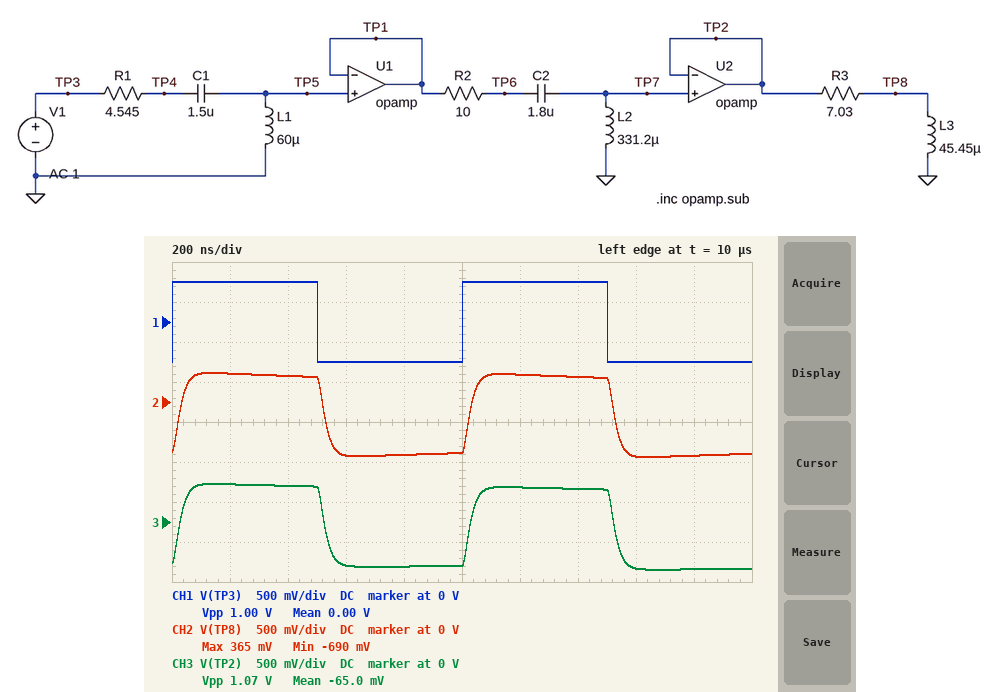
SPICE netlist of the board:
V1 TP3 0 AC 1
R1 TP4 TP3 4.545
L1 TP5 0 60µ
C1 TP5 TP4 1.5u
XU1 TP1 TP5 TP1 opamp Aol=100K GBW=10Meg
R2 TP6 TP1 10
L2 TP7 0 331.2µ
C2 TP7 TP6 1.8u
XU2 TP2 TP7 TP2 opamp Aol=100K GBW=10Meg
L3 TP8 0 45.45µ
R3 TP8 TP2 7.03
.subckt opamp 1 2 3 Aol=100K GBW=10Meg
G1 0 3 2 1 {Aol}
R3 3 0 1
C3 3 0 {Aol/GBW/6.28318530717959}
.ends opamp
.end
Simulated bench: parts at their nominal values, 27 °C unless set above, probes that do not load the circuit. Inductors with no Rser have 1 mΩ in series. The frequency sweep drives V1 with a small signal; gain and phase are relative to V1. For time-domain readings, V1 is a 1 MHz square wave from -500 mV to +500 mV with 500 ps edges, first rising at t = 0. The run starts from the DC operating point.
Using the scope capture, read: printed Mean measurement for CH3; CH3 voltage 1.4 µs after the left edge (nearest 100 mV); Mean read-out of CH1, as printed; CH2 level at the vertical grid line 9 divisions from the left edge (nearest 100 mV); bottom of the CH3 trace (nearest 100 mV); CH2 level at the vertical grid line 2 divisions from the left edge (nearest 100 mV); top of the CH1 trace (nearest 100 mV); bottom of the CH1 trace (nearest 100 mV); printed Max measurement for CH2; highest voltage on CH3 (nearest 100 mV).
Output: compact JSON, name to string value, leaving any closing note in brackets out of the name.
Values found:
{"printed Mean measurement for CH3": "-65.0 mV", "CH3 voltage 1.4 µs after the left edge": "400 mV", "Mean read-out of CH1, as printed": "0.00 V", "CH2 level at the vertical grid line 9 divisions from the left edge": "-700 mV", "bottom of the CH3 trace": "-600 mV", "CH2 level at the vertical grid line 2 divisions from the left edge": "300 mV", "top of the CH1 trace": "500 mV", "bottom of the CH1 trace": "-500 mV", "printed Max measurement for CH2": "365 mV", "highest voltage on CH3": "500 mV"}
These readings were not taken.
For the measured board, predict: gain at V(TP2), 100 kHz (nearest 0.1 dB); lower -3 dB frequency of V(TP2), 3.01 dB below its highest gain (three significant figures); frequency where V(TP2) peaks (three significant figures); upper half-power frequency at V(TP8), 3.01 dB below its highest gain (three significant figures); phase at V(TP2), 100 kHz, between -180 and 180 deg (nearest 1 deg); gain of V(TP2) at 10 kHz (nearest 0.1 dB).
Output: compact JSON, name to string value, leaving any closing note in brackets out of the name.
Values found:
{"gain at V(TP2), 100 kHz": "0.2 dB", "lower -3 dB frequency of V(TP2), 3.01 dB below its highest gain": "13.6 kHz", "frequency where V(TP2) peaks": "18.9 kHz", "upper half-power frequency at V(TP8), 3.01 dB below its highest gain": "6.10 MHz", "phase at V(TP2), 100 kHz, between -180 and 180 deg": "9 deg", "gain of V(TP2) at 10 kHz": "-4.3 dB"}
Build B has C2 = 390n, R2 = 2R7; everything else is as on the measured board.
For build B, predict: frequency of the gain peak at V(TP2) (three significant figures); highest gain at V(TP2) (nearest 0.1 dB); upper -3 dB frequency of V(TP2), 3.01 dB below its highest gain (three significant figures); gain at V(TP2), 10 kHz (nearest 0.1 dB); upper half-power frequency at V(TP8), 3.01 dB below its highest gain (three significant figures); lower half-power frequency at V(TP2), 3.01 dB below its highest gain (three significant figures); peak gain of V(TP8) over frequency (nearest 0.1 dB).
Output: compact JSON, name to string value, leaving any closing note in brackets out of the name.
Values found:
{"frequency of the gain peak at V(TP2)": "14.1 kHz", "highest gain at V(TP2)": "21.1 dB", "upper -3 dB frequency of V(TP2), 3.01 dB below its highest gain": "14.9 kHz", "gain at V(TP2), 10 kHz": "-6.5 dB", "upper half-power frequency at V(TP8), 3.01 dB below its highest gain": "15.0 kHz", "lower half-power frequency at V(TP2), 3.01 dB below its highest gain": "13.5 kHz", "peak gain of V(TP8) over frequency": "15.0 dB"}
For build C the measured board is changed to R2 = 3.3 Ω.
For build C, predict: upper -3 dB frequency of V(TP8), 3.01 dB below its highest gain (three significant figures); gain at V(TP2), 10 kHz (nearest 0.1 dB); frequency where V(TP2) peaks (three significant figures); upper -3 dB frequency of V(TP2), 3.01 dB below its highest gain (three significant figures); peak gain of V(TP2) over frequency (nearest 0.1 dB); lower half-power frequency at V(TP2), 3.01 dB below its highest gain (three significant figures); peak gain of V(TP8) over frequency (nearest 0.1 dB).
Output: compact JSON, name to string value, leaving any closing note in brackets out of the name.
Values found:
{"upper -3 dB frequency of V(TP8), 3.01 dB below its highest gain": "5.82 MHz", "gain at V(TP2), 10 kHz": "-2.3 dB", "frequency where V(TP2) peaks": "18.6 kHz", "upper -3 dB frequency of V(TP2), 3.01 dB below its highest gain": "38.0 kHz", "peak gain of V(TP2) over frequency": "4.5 dB", "lower half-power frequency at V(TP2), 3.01 dB below its highest gain": "13.2 kHz", "peak gain of V(TP8) over frequency": "0.5 dB"}
